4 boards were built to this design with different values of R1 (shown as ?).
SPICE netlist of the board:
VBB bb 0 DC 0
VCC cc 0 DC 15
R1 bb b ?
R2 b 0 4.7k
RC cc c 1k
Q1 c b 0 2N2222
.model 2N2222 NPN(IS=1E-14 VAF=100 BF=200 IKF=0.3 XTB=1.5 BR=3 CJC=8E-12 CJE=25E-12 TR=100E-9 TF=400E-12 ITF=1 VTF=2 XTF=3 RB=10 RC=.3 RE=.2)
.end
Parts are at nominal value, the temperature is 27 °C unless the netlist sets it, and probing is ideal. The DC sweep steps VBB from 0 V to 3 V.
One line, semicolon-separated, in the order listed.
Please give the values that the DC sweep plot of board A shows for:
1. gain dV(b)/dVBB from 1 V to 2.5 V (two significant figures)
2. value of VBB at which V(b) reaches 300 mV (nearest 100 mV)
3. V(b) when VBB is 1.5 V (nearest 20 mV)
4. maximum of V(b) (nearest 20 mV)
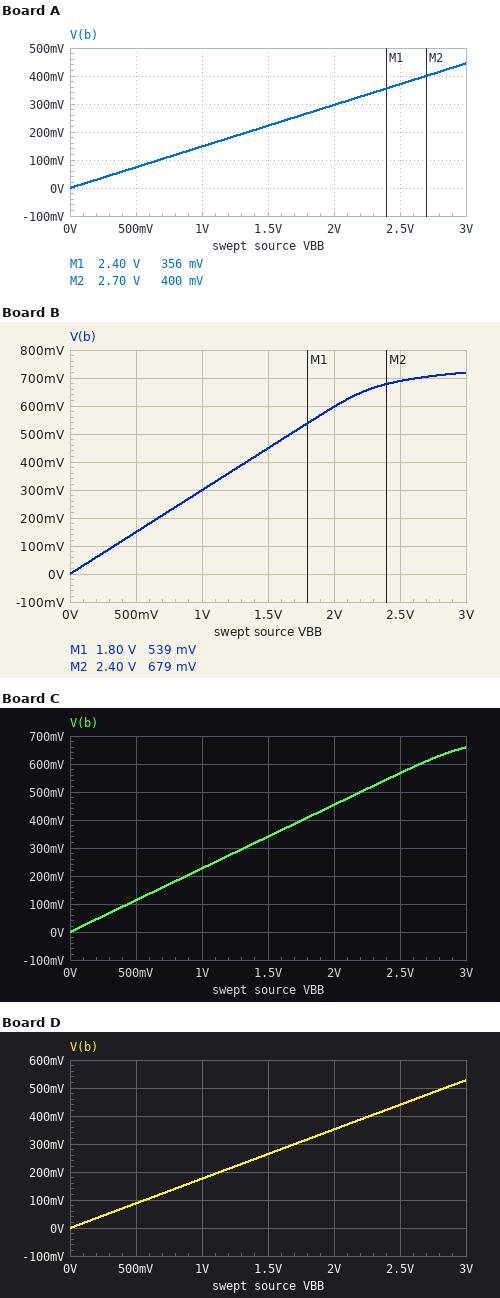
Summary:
0.15 V/V; 2.0 V; 220 mV; 440 mV
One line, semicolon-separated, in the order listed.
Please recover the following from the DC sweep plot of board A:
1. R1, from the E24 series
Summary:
27 kΩ
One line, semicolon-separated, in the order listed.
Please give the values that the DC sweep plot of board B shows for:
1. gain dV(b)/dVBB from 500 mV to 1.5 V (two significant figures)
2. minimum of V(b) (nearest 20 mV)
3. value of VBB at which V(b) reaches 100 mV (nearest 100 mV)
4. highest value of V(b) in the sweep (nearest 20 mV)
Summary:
0.30 V/V; 0 V; 300 mV; 720 mV
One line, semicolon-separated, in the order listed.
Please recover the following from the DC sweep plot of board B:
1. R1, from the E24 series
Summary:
11 kΩ
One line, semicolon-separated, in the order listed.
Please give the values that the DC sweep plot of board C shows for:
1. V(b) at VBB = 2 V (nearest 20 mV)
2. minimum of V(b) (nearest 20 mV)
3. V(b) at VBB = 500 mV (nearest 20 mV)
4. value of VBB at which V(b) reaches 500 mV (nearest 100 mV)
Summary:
460 mV; 0 V; 120 mV; 2.2 V
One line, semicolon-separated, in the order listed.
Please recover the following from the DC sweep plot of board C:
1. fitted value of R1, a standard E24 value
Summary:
16 kΩ
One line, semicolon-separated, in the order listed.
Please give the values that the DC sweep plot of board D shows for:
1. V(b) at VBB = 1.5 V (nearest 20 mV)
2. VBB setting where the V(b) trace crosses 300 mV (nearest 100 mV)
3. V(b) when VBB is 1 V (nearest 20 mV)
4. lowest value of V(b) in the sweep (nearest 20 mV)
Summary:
260 mV; 1.7 V; 180 mV; 0 V
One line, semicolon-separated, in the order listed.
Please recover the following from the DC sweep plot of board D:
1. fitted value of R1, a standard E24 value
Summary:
22 kΩ
